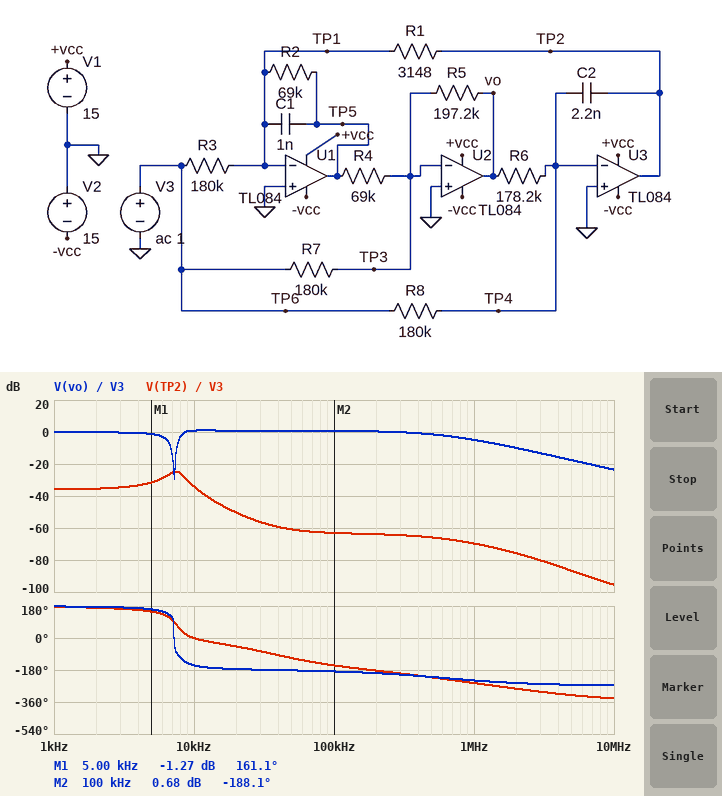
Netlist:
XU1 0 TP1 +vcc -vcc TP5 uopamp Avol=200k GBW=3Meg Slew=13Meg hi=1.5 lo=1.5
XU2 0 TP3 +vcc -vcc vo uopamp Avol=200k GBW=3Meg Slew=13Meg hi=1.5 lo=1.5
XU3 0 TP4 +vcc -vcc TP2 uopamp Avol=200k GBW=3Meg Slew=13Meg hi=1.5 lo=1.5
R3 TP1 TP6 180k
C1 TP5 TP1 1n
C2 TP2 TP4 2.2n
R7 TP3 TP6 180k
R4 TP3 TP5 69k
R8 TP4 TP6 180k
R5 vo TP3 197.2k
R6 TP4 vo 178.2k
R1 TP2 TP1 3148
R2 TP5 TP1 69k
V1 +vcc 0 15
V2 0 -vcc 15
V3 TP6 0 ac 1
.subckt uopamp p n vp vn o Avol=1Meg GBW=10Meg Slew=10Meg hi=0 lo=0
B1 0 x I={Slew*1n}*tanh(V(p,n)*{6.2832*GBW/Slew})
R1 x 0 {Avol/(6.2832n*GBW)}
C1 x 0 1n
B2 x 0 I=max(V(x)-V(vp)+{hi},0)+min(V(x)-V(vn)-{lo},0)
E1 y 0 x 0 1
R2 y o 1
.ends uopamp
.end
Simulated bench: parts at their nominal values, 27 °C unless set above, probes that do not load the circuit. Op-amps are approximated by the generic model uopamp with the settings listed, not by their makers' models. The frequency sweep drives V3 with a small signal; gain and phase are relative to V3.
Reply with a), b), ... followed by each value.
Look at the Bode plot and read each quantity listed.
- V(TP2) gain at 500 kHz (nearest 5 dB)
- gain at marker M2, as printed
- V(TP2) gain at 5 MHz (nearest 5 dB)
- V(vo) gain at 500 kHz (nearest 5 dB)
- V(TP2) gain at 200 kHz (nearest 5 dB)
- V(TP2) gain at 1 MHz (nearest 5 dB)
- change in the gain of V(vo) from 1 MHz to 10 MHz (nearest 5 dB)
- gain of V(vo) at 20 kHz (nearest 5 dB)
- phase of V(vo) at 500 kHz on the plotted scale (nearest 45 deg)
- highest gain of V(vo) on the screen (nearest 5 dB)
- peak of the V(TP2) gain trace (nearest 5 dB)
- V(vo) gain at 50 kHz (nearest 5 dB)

a) -65 dB
b) 0.68 dB
c) -85 dB
d) 0 dB
e) -65 dB
f) -70 dB
g) -20 dB
h) 0 dB
i) -225 deg
j) 0 dB
k) -25 dB
l) 0 dB
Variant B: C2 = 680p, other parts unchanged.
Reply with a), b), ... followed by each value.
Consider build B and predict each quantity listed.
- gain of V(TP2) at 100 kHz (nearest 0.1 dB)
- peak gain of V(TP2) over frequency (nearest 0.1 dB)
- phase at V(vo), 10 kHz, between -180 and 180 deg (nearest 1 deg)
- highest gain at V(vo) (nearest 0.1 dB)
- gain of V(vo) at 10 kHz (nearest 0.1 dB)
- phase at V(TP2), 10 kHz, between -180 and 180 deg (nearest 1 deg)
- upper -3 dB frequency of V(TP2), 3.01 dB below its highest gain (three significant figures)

a) -52.8 dB
b) -18.0 dB
c) 166 deg
d) 2.3 dB
e) -1.4 dB
f) 141 deg
g) 14.5 kHz
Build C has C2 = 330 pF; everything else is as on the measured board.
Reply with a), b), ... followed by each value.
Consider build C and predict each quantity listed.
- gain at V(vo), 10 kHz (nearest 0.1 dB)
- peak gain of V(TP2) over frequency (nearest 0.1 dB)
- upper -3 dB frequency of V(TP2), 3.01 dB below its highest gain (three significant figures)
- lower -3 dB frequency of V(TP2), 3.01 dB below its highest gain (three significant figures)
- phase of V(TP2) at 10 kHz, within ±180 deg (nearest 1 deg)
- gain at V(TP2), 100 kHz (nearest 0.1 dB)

a) -0.4 dB
b) -11.8 dB
c) 20.2 kHz
d) 18.9 kHz
e) 150 deg
f) -46.3 dB
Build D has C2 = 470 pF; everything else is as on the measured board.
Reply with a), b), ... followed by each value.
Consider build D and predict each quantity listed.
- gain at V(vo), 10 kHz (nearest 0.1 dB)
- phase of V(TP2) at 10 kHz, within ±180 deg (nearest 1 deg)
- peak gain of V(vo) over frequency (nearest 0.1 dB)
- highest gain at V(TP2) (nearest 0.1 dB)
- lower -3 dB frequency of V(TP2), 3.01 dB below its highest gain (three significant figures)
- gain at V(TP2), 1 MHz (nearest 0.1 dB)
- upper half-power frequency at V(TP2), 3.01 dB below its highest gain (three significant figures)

a) -0.7 dB
b) 147 deg
c) 3.4 dB
d) -15.2 dB
e) 15.5 kHz
f) -56.3 dB
g) 17.2 kHz
